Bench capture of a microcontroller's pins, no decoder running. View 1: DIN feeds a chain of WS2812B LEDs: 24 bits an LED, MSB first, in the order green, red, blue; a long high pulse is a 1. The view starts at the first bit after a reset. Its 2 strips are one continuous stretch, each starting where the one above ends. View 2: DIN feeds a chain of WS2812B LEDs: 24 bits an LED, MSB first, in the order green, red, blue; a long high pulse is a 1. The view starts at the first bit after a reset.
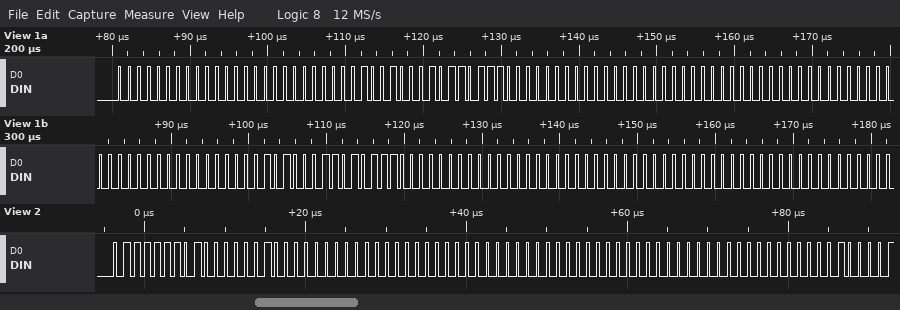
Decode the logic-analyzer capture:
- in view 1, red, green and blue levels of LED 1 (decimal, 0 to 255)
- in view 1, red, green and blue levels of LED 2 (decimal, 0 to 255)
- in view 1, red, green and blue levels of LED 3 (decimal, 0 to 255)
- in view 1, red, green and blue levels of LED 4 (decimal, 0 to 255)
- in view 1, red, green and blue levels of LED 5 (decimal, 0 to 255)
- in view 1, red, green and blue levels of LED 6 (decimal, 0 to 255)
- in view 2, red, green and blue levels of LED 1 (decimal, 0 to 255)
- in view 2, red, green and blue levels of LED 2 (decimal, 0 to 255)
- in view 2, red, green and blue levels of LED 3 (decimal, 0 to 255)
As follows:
0, 0, 0
183, 72, 0
0, 0, 0
0, 0, 0
174, 81, 0
0, 0, 0
129, 126, 0
0, 0, 0
0, 0, 0
